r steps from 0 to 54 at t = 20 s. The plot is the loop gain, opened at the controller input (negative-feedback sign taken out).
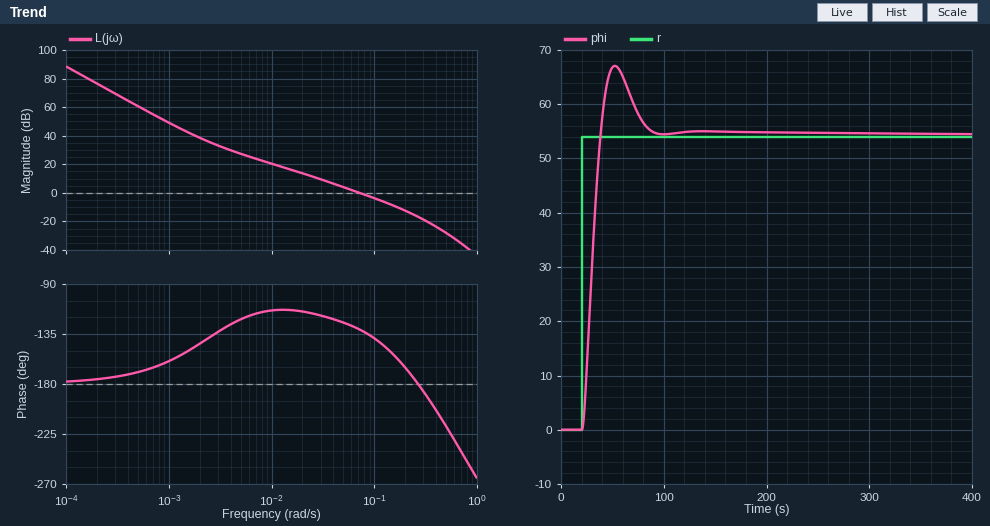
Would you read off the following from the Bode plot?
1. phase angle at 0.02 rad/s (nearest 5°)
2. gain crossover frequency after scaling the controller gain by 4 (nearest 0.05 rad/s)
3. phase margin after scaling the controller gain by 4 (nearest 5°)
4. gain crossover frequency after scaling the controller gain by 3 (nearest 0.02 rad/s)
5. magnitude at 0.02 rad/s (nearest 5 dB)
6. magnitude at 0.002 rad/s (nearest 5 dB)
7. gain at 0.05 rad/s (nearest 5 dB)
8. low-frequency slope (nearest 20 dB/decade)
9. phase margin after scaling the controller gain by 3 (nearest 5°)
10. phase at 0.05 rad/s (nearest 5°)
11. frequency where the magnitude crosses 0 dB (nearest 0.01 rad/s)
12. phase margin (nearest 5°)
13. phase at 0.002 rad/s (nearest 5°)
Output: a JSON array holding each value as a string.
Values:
["-115°", "0.20 rad/s", "15°", "0.16 rad/s", "15 dB", "40 dB", "5 dB", "-40 dB/decade", "25°", "-125°", "0.07 rad/s", "50°", "-145°"]
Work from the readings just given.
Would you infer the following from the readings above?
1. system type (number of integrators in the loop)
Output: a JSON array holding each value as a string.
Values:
["2"]
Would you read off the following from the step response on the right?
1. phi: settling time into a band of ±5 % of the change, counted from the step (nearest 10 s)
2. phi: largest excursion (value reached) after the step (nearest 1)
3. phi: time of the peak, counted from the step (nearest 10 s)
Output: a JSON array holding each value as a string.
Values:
["60 s", "67", "30 s"]
